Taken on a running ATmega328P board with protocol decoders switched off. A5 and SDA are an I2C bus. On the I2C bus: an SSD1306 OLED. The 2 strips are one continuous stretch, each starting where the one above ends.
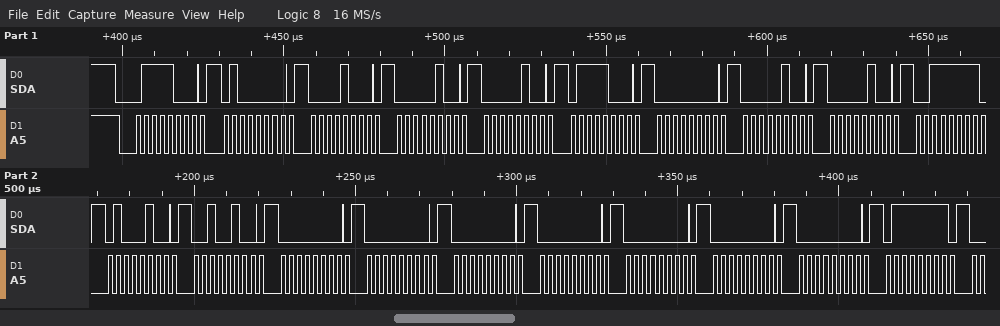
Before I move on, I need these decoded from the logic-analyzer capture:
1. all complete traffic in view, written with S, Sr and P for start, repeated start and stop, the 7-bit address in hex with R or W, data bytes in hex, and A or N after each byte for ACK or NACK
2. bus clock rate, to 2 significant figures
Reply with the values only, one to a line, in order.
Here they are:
S 3CW A 40 A 08 A 04 A 04 A 78 A 00 A 04 A 04 A 3F A 44 A 24 A 00 A 00 A 00 A 00 A 00 A 00 A 00 A 7F A
400 kHz
